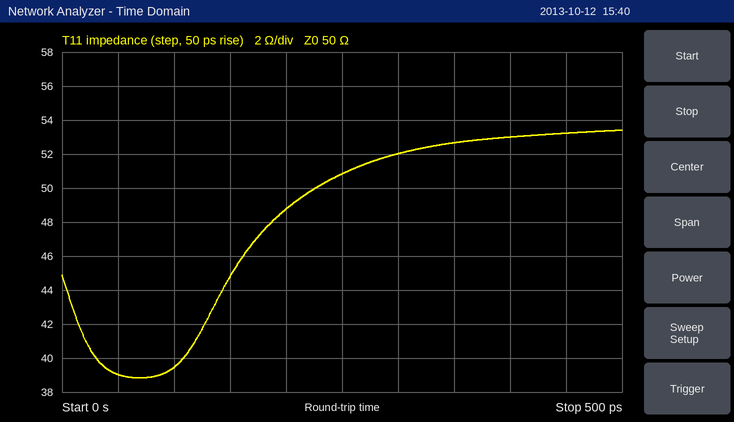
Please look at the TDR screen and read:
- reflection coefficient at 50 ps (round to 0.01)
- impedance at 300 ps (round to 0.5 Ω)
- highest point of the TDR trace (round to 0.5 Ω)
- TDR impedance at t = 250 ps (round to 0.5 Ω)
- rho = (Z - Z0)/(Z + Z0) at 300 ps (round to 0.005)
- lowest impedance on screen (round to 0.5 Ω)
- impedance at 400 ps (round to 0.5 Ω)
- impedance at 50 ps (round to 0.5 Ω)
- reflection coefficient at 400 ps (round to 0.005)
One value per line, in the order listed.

-0.12
52.0 Ω
53.5 Ω
51.0 Ω
+0.020
39.0 Ω
53.0 Ω
39.0 Ω
+0.030
